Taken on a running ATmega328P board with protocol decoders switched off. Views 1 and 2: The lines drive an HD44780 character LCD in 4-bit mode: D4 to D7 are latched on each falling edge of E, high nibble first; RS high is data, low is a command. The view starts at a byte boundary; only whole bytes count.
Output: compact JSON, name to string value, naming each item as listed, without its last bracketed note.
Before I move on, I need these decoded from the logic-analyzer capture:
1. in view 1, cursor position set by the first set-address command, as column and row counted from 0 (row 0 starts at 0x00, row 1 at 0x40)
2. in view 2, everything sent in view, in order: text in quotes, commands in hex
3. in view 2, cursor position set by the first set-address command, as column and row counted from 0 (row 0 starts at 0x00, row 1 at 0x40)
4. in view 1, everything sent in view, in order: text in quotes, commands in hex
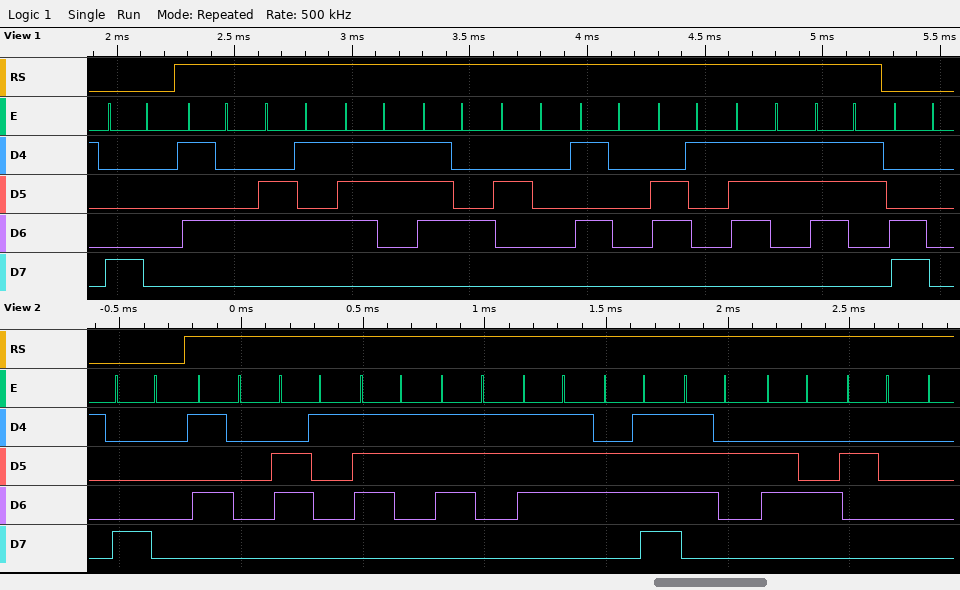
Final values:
{"in view 1, cursor position set by the first set-address command, as column and row counted from 0": "column 0, row 0", "in view 2, everything sent in view, in order: text in quotes, commands in hex": "0x80 \"Password \"", "in view 2, cursor position set by the first set-address command, as column and row counted from 0": "column 0, row 0", "in view 1, everything sent in view, in order: text in quotes, commands in hex": "0x80 \"Test Pass\" 0xC0"}
